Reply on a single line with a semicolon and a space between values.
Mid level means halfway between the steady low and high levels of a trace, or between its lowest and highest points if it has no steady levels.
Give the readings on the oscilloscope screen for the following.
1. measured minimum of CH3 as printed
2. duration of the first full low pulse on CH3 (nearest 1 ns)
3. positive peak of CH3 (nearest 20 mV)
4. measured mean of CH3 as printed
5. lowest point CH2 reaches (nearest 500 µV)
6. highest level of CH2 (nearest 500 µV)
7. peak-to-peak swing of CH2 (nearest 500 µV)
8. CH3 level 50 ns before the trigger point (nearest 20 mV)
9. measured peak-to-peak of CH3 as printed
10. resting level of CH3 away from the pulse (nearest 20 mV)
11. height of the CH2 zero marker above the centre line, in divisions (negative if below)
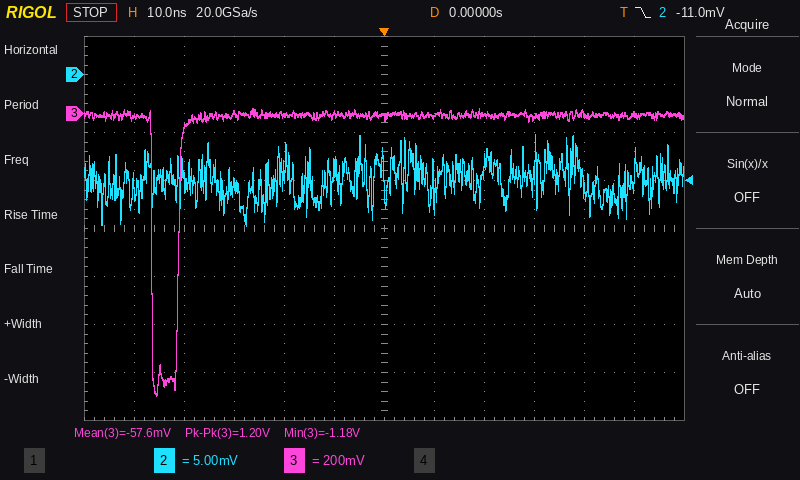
-1.18 V; 5 ns; 20 mV; -57.6 mV; -15.5 mV; -6.0 mV; 9.5 mV; -20 mV; 1.20 V; 0 mV; +3.2 div
